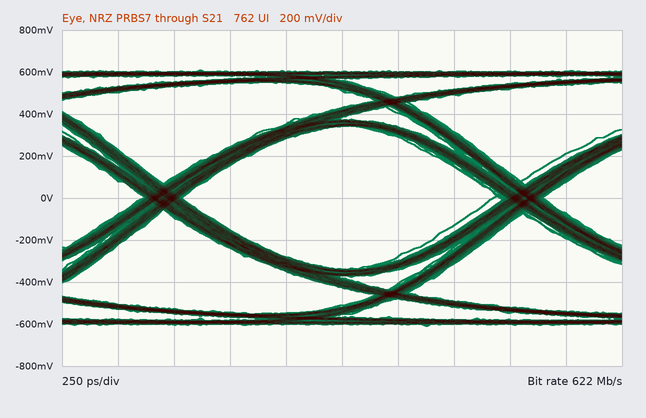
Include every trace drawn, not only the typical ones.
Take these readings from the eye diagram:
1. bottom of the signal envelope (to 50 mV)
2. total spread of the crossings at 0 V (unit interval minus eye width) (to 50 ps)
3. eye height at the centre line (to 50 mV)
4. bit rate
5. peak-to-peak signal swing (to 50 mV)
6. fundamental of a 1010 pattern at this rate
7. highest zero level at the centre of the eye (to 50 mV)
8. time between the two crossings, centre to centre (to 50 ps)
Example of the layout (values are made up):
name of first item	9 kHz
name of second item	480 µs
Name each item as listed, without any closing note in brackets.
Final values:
bottom of the signal envelope	-600 mV
total spread of the crossings at 0 V (unit interval minus eye width)	200 ps
eye height at the centre line	700 mV
bit rate	622 Mb/s
peak-to-peak signal swing	1.20 V
fundamental of a 1010 pattern at this rate	311 MHz
highest zero level at the centre of the eye	-350 mV
time between the two crossings, centre to centre	1.60 ns
